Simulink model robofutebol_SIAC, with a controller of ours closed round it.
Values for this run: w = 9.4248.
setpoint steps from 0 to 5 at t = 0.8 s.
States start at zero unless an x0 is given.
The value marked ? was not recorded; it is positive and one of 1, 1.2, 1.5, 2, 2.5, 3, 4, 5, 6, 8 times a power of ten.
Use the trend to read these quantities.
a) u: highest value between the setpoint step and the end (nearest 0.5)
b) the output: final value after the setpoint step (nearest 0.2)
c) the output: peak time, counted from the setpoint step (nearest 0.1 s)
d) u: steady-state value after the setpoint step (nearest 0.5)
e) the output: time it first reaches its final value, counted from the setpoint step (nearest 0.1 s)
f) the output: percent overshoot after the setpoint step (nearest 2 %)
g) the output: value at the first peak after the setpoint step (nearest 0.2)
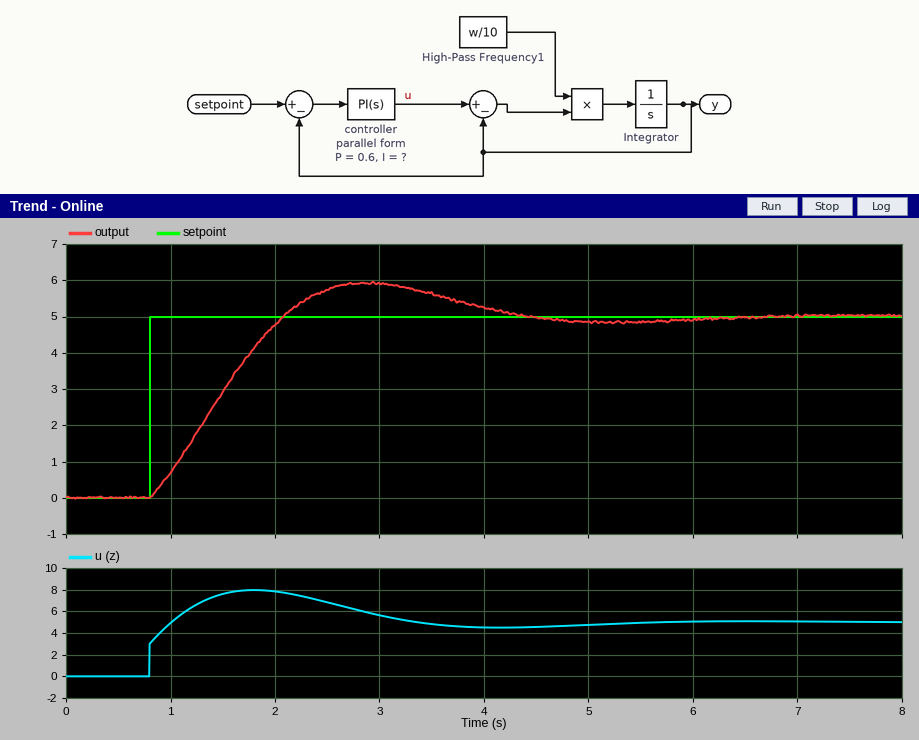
8.0
5.0
2.1 s
5.0
1.3 s
18 %
6.0
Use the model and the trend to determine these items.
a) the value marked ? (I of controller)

2.5
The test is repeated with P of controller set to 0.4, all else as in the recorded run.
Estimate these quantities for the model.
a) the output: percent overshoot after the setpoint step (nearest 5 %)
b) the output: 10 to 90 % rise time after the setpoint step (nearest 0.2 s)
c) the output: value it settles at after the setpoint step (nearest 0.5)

25 %
1.0 s
5.0
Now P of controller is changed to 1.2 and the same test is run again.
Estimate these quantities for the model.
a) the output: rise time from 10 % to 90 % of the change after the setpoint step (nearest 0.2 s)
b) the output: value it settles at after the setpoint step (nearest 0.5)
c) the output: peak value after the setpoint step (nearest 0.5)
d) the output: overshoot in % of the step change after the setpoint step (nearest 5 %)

1.0 s
5.0
5.5
10 %
